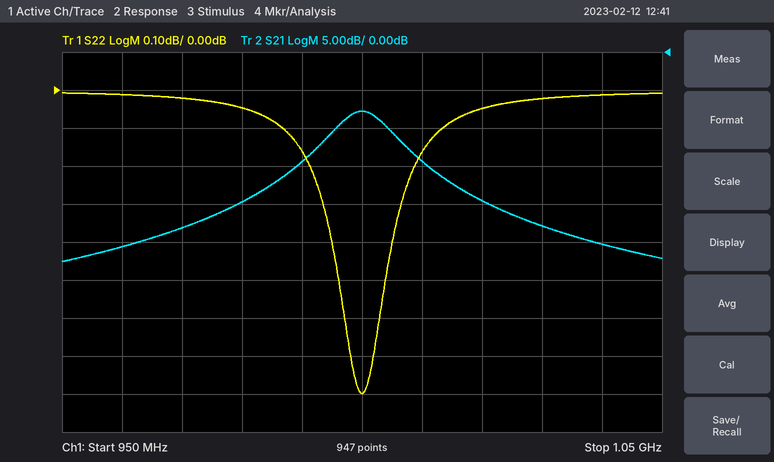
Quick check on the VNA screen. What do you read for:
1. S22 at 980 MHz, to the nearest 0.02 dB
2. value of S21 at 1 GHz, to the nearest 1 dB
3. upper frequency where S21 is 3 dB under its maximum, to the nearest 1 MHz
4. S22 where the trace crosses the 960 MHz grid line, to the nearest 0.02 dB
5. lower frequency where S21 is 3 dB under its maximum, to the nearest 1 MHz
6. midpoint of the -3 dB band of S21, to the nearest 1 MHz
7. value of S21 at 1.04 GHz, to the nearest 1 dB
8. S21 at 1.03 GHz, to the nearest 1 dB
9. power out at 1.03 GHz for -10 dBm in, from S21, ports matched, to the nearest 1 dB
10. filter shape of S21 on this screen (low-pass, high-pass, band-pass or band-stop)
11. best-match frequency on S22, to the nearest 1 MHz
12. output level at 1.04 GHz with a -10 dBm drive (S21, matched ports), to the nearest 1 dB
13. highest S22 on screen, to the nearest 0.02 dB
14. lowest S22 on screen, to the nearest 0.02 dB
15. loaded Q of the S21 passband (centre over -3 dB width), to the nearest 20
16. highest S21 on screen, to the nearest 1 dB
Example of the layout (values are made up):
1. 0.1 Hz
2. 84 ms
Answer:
1. -0.04 dB
2. -8 dB
3. 1.005 GHz
4. -0.02 dB
5. 995 MHz
6. 1.000 GHz
7. -25 dB
8. -23 dB
9. -33 dBm
10. band-pass
11. 1.000 GHz
12. -35 dBm
13. 0.00 dB
14. -0.80 dB
15. 100
16. -8 dB
